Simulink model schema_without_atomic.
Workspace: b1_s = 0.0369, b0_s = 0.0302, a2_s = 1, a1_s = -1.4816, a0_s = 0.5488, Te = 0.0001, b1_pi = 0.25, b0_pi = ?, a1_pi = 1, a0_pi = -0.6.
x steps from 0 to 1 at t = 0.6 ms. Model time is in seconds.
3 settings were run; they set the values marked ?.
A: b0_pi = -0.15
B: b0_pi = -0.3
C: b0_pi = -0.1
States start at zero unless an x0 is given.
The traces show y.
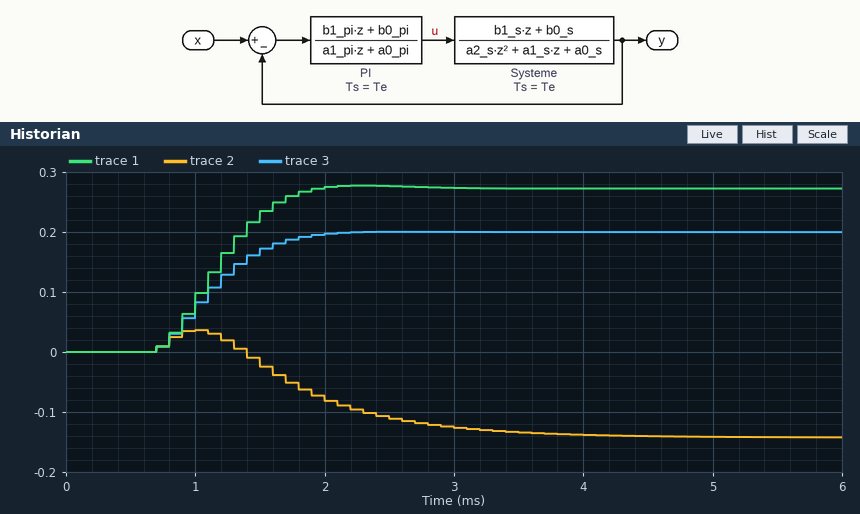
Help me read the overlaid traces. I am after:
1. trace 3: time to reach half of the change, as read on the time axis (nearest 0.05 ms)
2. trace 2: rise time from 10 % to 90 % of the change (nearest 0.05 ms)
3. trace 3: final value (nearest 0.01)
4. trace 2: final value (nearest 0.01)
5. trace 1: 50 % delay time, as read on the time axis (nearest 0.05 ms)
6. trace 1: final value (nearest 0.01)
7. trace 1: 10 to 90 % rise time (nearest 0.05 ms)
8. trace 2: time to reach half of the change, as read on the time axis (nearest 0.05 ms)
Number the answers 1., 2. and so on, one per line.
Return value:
1. 1.10 ms
2. 1.60 ms
3. 0.20
4. -0.14
5. 1.20 ms
6. 0.27
7. 0.80 ms
8. 1.90 ms
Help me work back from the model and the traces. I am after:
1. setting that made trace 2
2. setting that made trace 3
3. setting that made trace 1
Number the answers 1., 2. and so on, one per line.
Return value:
1. B
2. A
3. C
